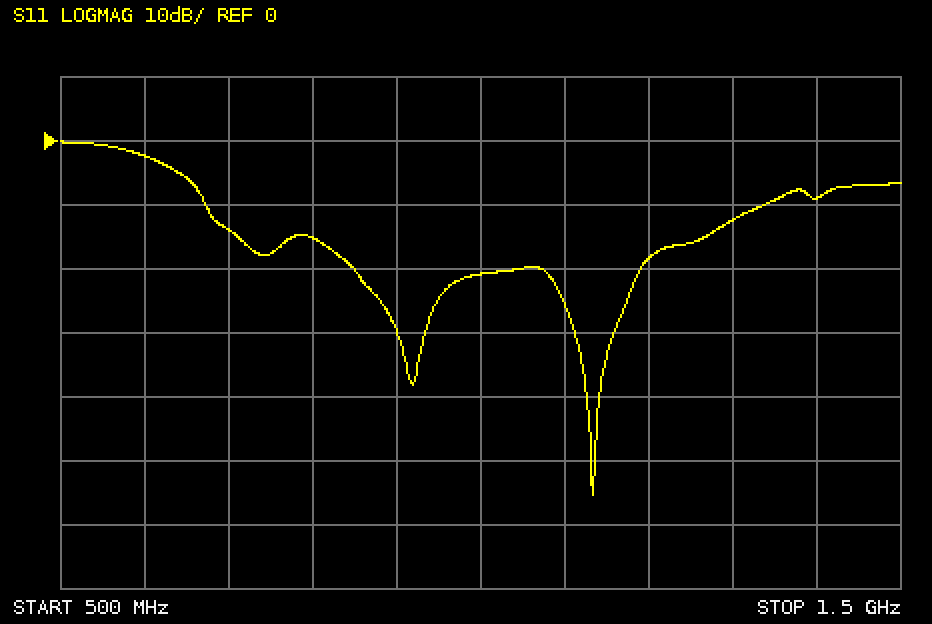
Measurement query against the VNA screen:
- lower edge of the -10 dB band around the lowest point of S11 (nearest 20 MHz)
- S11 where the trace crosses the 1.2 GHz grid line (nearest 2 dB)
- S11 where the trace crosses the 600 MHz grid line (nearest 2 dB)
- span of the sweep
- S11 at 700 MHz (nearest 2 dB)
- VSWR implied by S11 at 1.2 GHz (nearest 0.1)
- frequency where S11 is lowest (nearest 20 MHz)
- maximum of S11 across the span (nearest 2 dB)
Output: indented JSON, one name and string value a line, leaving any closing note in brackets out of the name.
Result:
{
  "lower edge of the -10 dB band around the lowest point of S11": "680 MHz",
  "S11 where the trace crosses the 1.2 GHz grid line": "-18 dB",
  "S11 where the trace crosses the 600 MHz grid line": "-2 dB",
  "span of the sweep": "1 GHz",
  "S11 at 700 MHz": "-14 dB",
  "VSWR implied by S11 at 1.2 GHz": "1.3",
  "frequency where S11 is lowest": "1.14 GHz",
  "maximum of S11 across the span": "0 dB"
}
